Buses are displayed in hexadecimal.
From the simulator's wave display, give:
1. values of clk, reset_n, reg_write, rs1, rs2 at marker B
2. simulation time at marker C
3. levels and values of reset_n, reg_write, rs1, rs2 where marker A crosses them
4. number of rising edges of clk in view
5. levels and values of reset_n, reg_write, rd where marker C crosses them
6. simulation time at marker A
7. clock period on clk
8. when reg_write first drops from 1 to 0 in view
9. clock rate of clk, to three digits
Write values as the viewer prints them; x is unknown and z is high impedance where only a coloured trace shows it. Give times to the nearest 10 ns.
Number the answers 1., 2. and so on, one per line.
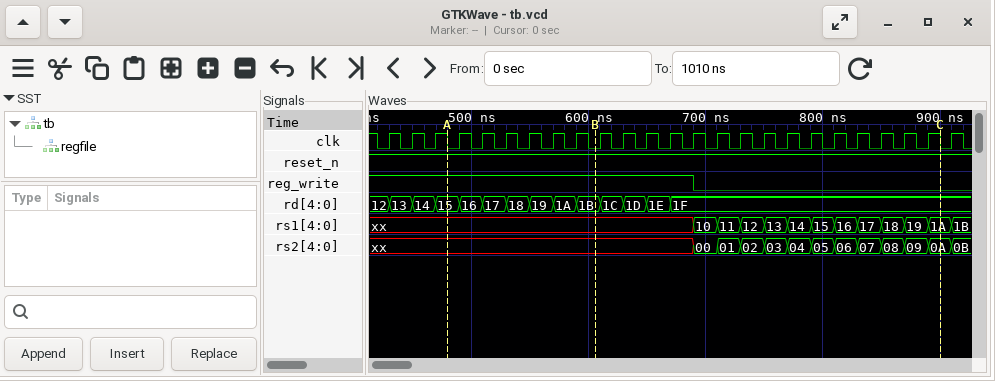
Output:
1. clk=0, reset_n=1, reg_write=1, rs1=xx, rs2=xx
2. 900 ns
3. reset_n=1, reg_write=1, rs1=xx, rs2=xx
4. 25
5. reset_n=1, reg_write=0, rd=1F
6. 480 ns
7. 20 ns
8. 690 ns
9. 50.0 MHz
